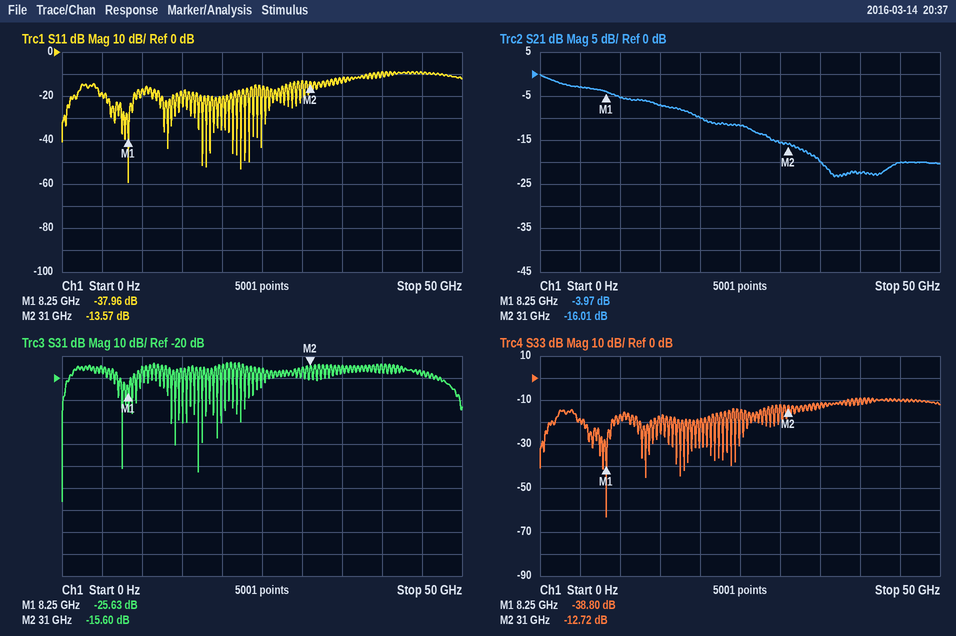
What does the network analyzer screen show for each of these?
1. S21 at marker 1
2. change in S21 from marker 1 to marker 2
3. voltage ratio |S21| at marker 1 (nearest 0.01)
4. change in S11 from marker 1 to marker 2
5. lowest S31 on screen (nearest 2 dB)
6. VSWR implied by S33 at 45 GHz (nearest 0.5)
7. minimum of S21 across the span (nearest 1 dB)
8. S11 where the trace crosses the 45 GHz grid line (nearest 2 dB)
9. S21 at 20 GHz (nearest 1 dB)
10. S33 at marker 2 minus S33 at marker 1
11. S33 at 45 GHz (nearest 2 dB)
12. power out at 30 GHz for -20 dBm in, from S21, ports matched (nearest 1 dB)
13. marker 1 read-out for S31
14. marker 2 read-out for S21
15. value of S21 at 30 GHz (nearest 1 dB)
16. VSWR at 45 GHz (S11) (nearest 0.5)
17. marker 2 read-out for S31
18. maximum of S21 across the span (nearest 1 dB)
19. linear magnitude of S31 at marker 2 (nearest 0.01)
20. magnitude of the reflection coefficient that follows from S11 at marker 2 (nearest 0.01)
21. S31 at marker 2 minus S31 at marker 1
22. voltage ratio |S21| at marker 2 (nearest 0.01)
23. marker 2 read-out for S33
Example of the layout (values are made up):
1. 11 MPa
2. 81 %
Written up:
1. -3.97 dB
2. -12.04 dB
3. 0.63
4. 24.39 dB
5. -76 dB
6. 2.0
7. -23 dB
8. -10 dB
9. -10 dB
10. 26.08 dB
11. -10 dB
12. -36 dBm
13. -25.63 dB
14. -16.01 dB
15. -16 dB
16. 2.0
17. -15.60 dB
18. 0 dB
19. 0.17
20. 0.21
21. 10.03 dB
22. 0.16
23. -12.72 dB
